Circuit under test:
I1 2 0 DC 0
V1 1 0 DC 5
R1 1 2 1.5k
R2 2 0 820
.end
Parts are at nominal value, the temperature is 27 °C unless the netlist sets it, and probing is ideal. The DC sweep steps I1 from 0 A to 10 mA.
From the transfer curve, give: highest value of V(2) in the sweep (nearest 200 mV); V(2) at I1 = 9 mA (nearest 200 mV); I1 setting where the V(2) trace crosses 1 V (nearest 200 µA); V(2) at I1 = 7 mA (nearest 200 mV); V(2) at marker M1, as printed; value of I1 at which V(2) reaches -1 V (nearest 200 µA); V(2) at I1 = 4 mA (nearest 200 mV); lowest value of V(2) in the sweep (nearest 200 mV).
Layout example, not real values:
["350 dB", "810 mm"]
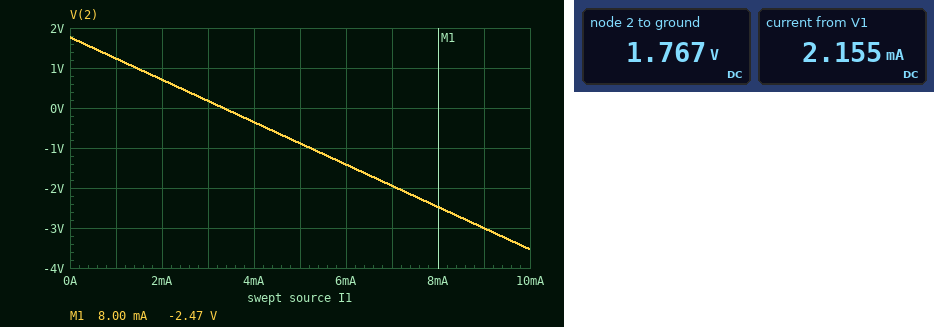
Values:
["1.8 V", "-3.0 V", "1.4 mA", "-2.0 V", "-2.47 V", "5.2 mA", "-400 mV", "-3.6 V"]
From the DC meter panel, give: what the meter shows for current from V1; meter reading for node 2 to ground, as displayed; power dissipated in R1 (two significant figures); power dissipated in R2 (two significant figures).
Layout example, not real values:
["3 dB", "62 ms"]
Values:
["2.155 mA", "1.767 V", "7.0 mW", "3.8 mW"]
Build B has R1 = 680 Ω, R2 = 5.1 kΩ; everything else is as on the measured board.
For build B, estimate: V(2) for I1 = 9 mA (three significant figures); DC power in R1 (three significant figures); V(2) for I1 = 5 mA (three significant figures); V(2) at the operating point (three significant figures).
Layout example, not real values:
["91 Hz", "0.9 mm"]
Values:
["-988 mV", "509 µW", "1.41 V", "4.41 V"]
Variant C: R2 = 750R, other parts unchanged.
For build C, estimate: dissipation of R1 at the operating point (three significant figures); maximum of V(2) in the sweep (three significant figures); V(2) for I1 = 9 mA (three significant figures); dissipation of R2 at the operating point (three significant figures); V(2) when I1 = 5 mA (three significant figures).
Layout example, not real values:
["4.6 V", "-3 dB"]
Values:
["7.41 mW", "1.67 V", "-2.83 V", "3.70 mW", "-833 mV"]
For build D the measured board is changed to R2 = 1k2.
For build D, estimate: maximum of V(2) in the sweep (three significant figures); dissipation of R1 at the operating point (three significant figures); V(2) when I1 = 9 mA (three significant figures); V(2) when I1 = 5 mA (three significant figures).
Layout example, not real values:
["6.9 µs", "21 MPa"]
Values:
["2.22 V", "5.14 mW", "-3.78 V", "-1.11 V"]
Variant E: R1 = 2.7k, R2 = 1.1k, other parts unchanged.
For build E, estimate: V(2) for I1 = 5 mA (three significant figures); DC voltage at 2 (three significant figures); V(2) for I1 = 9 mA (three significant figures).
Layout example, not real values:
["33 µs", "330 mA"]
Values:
["-2.46 V", "1.45 V", "-5.59 V"]
